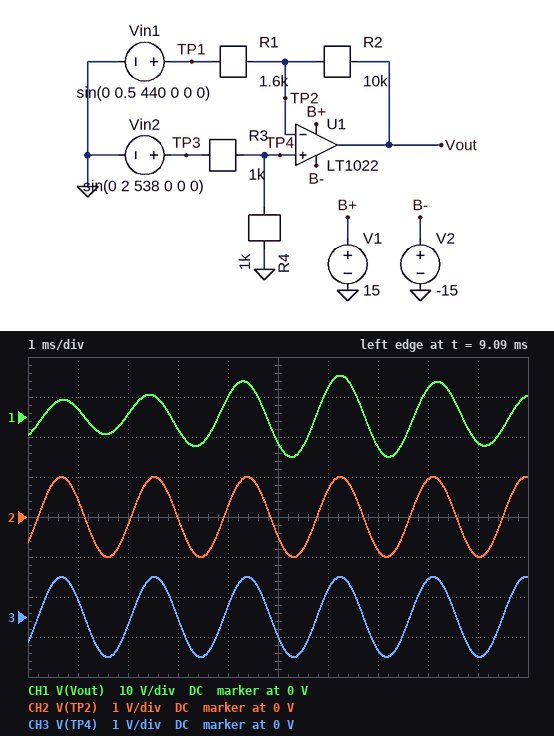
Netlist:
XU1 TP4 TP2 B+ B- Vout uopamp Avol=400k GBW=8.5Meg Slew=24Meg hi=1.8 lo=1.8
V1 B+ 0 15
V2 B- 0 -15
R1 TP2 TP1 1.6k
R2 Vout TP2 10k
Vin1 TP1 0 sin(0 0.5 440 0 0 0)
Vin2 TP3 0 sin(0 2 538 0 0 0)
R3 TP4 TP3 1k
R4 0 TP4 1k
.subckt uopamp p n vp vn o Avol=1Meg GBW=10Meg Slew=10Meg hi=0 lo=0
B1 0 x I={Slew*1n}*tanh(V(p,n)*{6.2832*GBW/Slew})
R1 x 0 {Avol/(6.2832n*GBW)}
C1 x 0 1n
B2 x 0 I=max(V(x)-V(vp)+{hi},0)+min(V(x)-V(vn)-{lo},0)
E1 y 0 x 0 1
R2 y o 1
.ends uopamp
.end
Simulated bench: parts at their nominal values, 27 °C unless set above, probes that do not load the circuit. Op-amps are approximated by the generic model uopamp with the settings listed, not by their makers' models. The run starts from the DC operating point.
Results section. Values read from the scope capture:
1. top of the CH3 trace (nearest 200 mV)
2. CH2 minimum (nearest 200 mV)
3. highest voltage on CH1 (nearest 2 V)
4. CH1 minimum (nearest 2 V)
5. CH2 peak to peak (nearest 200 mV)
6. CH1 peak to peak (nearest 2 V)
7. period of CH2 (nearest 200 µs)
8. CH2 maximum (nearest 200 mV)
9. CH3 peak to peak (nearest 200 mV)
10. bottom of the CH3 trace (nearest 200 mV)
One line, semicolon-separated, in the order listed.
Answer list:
1.0 V; -1.0 V; 10 V; -10 V; 2.0 V; 20 V; 1.8 ms; 1.0 V; 2.0 V; -1.0 V
